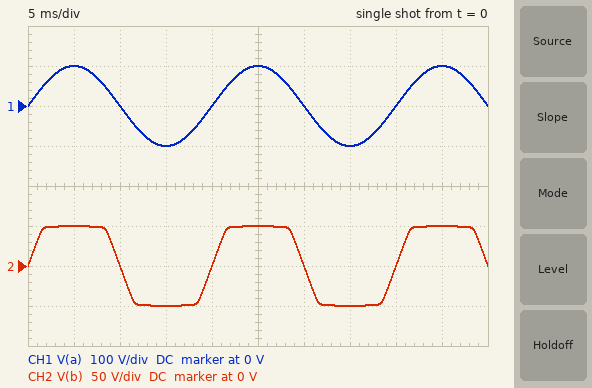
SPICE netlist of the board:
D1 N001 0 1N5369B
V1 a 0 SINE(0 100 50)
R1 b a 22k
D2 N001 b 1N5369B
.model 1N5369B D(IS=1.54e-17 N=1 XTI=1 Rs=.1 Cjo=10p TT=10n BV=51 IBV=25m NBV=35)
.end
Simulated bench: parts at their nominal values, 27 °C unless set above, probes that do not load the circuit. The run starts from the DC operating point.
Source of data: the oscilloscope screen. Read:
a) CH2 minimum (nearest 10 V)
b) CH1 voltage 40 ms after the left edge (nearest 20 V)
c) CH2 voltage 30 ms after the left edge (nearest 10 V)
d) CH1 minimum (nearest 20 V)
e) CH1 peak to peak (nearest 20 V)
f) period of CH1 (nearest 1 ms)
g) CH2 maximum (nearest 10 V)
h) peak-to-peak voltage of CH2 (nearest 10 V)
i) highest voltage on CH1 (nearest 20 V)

-50 V
0 V
0 V
-100 V
200 V
20 ms
50 V
100 V
100 V
